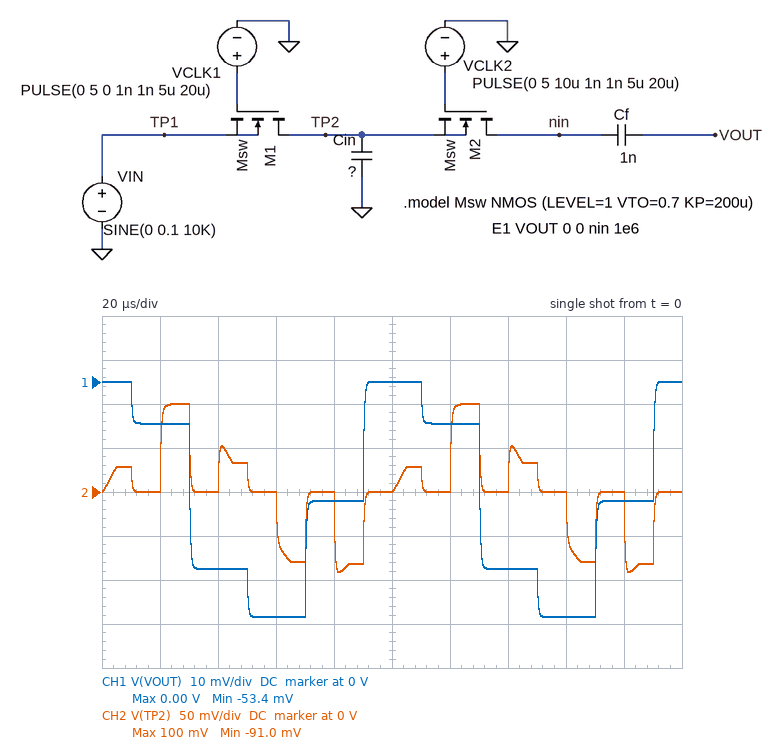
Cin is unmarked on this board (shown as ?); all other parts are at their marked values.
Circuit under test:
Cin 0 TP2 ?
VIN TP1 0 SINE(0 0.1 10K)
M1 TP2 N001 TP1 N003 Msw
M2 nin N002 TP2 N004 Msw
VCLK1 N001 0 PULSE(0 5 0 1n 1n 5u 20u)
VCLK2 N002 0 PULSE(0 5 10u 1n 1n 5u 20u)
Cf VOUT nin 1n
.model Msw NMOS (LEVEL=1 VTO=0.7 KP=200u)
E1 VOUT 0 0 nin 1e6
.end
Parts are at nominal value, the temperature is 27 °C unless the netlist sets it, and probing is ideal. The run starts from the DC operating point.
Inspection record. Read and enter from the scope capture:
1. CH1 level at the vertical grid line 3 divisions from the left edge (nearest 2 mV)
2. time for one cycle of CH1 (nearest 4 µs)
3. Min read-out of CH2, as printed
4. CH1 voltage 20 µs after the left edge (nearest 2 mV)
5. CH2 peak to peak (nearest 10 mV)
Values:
-54 mV
100 µs
-91.0 mV
-10 mV
190 mV
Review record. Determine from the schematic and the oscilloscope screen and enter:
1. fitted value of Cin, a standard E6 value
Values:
330 pF
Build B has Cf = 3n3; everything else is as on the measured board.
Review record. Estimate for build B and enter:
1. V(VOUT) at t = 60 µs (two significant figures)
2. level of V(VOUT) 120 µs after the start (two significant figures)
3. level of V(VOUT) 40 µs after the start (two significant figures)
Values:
-16 mV
-2.9 mV
-13 mV
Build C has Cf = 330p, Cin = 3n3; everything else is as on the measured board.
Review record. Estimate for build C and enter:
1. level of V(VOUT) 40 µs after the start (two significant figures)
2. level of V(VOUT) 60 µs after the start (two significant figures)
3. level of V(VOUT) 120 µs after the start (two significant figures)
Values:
-630 mV
-890 mV
-89 mV
